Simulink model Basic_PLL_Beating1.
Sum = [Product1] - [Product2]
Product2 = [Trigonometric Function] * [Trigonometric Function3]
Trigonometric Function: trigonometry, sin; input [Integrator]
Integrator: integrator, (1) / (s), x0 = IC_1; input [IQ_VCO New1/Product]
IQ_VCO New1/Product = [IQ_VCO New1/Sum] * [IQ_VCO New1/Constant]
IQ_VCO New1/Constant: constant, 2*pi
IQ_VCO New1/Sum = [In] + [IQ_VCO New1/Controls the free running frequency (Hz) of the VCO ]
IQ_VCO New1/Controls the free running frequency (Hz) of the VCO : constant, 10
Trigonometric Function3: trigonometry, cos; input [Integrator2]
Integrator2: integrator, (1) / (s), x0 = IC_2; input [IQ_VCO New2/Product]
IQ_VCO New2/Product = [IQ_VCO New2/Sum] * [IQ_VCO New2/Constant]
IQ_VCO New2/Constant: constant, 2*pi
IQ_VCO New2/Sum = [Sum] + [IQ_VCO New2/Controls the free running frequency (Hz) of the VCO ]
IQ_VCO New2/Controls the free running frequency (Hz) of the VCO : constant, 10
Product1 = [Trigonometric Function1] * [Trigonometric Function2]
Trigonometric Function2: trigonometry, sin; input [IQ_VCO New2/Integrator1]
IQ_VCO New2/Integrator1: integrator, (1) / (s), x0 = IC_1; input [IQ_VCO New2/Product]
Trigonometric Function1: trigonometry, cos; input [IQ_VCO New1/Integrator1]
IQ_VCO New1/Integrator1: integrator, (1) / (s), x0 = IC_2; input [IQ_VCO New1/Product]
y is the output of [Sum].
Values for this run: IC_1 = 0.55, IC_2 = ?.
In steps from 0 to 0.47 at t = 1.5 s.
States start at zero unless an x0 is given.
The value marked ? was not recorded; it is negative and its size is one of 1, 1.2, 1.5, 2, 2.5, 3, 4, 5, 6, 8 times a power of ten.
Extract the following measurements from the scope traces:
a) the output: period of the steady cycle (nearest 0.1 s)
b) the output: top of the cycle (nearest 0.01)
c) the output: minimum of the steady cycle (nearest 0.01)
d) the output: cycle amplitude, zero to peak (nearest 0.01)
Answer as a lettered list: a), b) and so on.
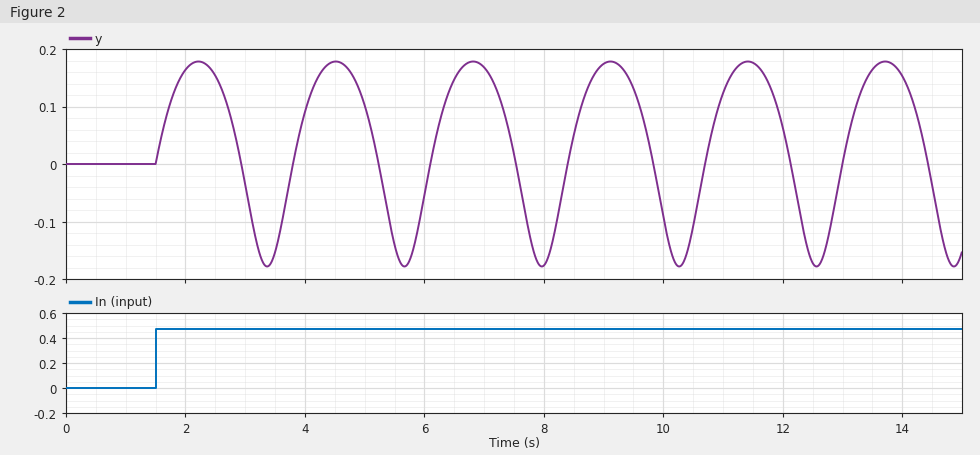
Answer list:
a) 2.3 s
b) 0.18
c) -0.18
d) 0.18
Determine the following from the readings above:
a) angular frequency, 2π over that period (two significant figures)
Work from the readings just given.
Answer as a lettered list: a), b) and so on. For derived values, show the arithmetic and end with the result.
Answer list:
a) 2π / 2.3 = 2.7 rad/s
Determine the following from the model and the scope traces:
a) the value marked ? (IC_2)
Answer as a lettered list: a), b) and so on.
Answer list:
a) -1.2
